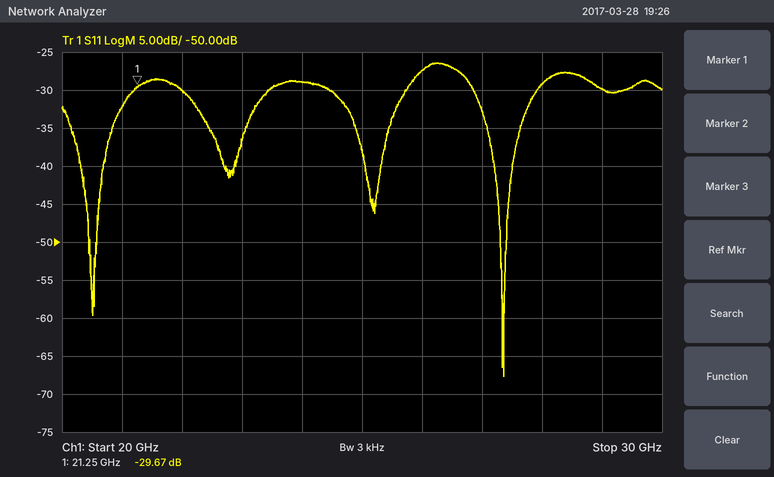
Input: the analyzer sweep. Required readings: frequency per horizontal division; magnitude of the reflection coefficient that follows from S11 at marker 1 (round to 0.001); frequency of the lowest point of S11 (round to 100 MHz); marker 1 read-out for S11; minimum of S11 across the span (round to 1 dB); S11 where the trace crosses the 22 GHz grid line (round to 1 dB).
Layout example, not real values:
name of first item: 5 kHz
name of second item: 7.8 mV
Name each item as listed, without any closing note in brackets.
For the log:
frequency per horizontal division: 1 GHz
magnitude of the reflection coefficient that follows from S11 at marker 1: 0.033
frequency of the lowest point of S11: 27.4 GHz
marker 1 read-out for S11: -29.67 dB
minimum of S11 across the span: -68 dB
S11 where the trace crosses the 22 GHz grid line: -30 dB
